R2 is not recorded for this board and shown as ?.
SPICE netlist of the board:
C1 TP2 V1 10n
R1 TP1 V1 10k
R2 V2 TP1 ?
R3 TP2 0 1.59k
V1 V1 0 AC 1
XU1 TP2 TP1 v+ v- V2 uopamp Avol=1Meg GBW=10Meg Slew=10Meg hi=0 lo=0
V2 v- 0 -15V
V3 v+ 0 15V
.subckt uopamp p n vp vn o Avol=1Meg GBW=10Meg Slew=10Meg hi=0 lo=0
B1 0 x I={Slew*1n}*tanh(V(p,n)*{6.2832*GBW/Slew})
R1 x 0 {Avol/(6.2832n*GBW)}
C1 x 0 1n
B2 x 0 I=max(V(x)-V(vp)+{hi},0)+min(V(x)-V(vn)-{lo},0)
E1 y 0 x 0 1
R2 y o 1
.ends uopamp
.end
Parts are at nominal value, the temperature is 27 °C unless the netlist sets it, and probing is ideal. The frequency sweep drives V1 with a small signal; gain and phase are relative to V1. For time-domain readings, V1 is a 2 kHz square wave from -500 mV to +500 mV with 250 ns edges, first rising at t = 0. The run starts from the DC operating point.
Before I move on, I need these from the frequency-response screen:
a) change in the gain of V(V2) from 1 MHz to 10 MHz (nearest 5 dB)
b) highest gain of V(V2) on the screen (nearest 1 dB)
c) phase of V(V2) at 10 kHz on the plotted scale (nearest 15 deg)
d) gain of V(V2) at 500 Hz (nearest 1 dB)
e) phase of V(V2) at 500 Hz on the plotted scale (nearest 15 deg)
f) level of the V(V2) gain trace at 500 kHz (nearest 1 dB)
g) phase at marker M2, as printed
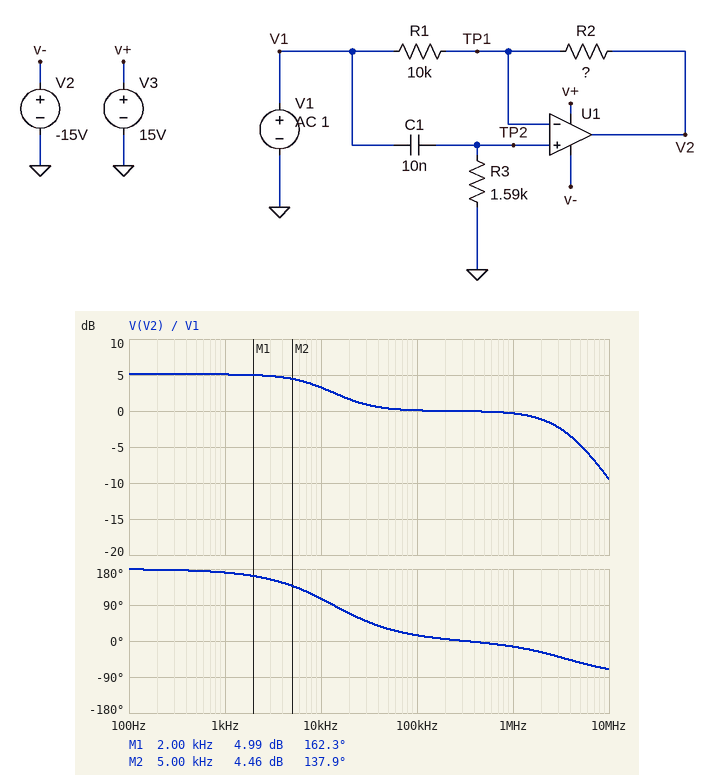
-10 dB
5 dB
105 deg
5 dB
180 deg
0 dB
137.9 deg
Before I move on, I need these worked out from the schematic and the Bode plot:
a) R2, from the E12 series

18 kΩ
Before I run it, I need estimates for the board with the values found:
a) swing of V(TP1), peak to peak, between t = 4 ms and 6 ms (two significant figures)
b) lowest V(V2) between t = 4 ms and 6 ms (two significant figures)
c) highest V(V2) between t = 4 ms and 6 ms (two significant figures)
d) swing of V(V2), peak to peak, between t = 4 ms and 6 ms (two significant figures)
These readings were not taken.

2.0 V
-1.9 V
1.9 V
3.7 V
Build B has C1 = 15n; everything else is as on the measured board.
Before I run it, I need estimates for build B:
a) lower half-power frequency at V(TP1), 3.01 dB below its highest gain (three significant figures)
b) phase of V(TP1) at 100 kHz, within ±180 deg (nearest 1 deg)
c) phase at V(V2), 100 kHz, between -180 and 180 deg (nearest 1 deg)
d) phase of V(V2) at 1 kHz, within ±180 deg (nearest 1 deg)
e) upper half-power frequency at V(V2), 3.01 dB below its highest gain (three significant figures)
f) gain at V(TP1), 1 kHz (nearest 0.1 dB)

6.65 kHz
3 deg
9 deg
167 deg
10.8 kHz
-16.6 dB
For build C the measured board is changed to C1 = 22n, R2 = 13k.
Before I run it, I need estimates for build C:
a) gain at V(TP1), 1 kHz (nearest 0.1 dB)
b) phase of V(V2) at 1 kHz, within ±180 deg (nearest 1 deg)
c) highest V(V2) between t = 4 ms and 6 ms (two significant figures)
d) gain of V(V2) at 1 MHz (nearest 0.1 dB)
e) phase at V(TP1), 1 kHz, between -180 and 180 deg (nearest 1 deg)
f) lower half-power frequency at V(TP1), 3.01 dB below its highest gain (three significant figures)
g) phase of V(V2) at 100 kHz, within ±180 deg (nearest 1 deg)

-13.4 dB
158 deg
1.6 V
-0.2 dB
78 deg
4.54 kHz
5 deg
